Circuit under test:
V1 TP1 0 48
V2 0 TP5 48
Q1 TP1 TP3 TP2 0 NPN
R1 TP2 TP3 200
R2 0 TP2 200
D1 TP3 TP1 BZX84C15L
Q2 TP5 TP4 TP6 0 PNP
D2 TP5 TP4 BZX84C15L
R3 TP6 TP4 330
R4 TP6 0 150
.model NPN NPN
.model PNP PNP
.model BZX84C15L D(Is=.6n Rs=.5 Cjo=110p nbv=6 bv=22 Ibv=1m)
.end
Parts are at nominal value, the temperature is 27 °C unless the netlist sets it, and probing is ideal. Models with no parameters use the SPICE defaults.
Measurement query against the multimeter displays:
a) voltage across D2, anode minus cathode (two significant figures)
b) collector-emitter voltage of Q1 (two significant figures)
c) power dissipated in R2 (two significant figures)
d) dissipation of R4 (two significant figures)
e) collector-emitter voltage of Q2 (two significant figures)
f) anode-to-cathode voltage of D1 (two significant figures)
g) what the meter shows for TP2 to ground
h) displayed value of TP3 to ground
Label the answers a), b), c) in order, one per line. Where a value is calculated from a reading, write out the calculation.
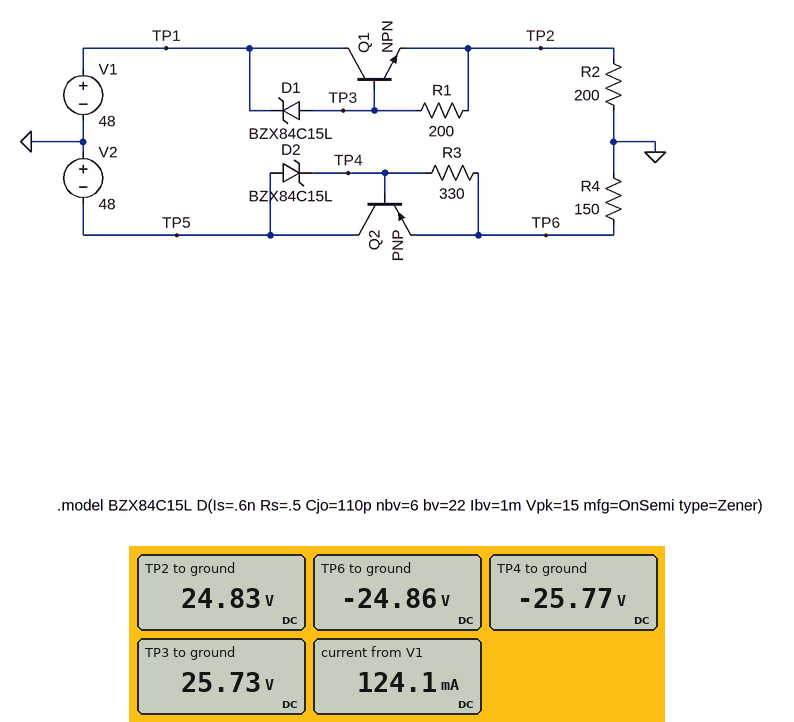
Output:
a) -48 V - (-25.77 V) = -22 V
b) 48 V - 24.83 V = 23 V
c) (24.83 V)^2 / 200 Ω = 3.1 W
d) (0 V - (-24.86 V))^2 / 150 Ω = 4.1 W
e) -48 V - (-24.86 V) = -23 V
f) 25.73 V - 48 V = -22 V
g) 24.83 V
h) 25.73 V
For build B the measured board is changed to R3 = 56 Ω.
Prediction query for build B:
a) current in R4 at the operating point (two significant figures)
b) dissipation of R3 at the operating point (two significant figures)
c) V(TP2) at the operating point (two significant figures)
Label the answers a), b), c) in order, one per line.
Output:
a) 160 mA
b) 15 mW
c) 25 V
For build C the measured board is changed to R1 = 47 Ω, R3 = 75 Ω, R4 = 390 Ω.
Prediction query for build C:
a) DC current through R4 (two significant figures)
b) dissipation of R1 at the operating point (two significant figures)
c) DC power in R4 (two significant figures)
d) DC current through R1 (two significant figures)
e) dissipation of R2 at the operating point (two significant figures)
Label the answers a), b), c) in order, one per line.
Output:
a) 63 mA
b) 17 mW
c) 1.6 W
d) 19 mA
e) 3.0 W
